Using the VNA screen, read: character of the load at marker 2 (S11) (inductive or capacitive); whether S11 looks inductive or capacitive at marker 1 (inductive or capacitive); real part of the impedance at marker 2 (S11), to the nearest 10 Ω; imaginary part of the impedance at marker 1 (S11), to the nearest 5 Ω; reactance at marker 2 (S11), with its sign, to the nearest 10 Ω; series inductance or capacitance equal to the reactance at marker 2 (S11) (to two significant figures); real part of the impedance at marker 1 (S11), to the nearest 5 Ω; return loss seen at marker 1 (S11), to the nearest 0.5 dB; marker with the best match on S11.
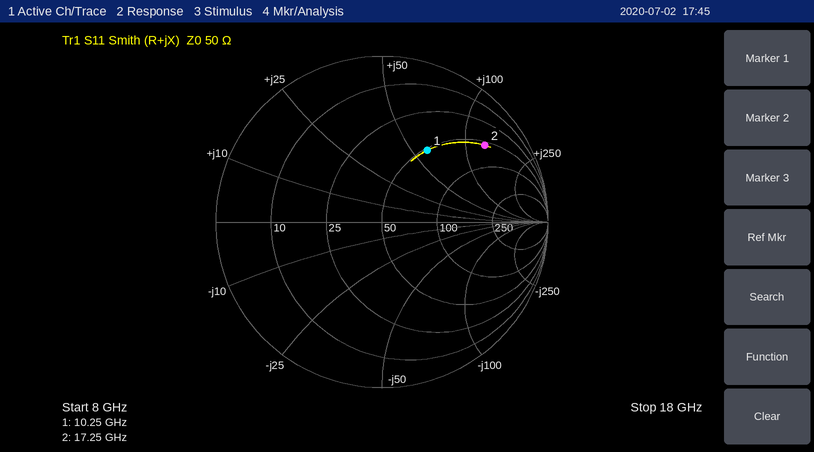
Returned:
inductive
inductive
60 Ω
+60 Ω
+130 Ω
1.2 nH
50 Ω
6.0 dB
marker 1
